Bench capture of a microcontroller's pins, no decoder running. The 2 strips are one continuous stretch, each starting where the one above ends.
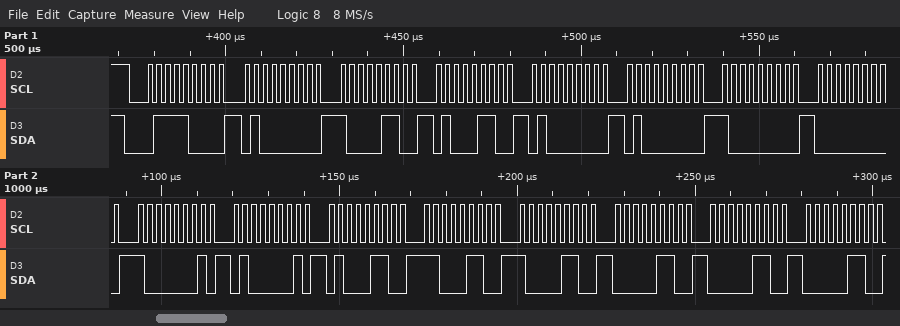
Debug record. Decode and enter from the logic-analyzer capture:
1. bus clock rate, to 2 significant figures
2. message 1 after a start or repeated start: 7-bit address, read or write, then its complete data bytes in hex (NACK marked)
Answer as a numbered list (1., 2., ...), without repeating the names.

1. 400 kHz
2. 0x3C write: 40 86 46 40 40 80 00 81 41 46 C6 86 06 06 06
